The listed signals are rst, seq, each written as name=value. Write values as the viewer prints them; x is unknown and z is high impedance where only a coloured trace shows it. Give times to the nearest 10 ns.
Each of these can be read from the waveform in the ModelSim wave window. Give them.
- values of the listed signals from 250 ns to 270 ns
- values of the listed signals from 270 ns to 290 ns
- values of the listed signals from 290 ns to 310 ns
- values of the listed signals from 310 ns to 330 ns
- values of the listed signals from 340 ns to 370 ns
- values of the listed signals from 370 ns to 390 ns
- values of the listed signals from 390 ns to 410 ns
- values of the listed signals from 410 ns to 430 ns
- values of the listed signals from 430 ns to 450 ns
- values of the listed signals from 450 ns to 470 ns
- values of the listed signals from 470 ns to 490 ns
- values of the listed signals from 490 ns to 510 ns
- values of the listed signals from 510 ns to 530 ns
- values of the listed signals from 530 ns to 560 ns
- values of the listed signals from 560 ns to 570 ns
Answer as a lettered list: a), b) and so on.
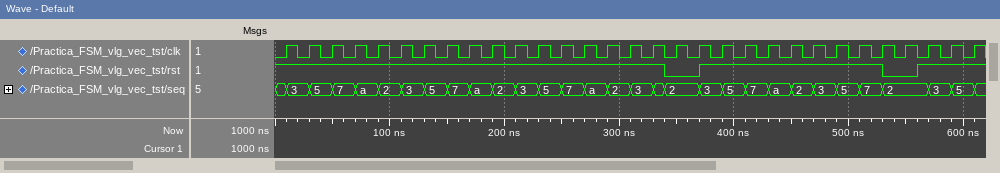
a) rst=1, seq=7
b) rst=1, seq=a
c) rst=1, seq=2
d) rst=1, seq=3
e) rst=0, seq=2
f) rst=1, seq=3
g) rst=1, seq=5
h) rst=1, seq=7
i) rst=1, seq=a
j) rst=1, seq=2
k) rst=1, seq=3
l) rst=1, seq=5
m) rst=1, seq=7
n) rst=0, seq=2
o) rst=1, seq=2
